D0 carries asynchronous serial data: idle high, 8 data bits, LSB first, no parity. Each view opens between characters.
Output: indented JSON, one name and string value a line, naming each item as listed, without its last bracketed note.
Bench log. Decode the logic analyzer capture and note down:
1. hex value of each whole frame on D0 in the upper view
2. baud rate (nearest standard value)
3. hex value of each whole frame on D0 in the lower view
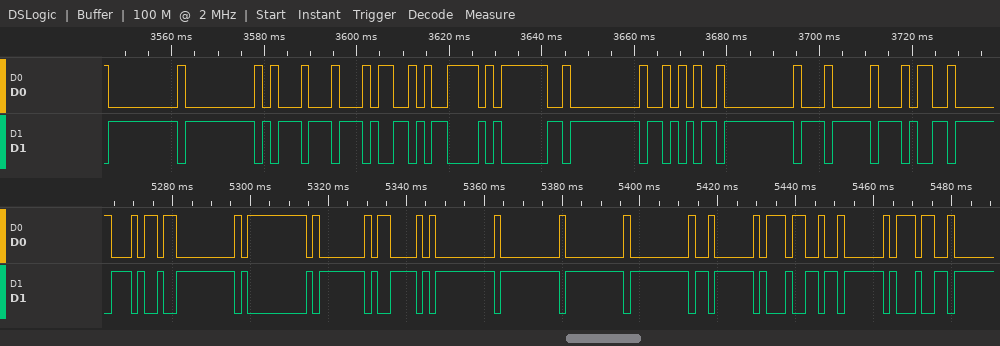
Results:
{
  "hex value of each whole frame on D0 in the upper view": "00, 00, 11, 34, 79, 3F, 00, 2A, 00, 04, 34",
  "baud rate": "600 baud",
  "hex value of each whole frame on D0 in the lower view": "B4, 00, FF, 01, 43, 00, 00, 00, 00, 02, 37, 02, 37"
}
